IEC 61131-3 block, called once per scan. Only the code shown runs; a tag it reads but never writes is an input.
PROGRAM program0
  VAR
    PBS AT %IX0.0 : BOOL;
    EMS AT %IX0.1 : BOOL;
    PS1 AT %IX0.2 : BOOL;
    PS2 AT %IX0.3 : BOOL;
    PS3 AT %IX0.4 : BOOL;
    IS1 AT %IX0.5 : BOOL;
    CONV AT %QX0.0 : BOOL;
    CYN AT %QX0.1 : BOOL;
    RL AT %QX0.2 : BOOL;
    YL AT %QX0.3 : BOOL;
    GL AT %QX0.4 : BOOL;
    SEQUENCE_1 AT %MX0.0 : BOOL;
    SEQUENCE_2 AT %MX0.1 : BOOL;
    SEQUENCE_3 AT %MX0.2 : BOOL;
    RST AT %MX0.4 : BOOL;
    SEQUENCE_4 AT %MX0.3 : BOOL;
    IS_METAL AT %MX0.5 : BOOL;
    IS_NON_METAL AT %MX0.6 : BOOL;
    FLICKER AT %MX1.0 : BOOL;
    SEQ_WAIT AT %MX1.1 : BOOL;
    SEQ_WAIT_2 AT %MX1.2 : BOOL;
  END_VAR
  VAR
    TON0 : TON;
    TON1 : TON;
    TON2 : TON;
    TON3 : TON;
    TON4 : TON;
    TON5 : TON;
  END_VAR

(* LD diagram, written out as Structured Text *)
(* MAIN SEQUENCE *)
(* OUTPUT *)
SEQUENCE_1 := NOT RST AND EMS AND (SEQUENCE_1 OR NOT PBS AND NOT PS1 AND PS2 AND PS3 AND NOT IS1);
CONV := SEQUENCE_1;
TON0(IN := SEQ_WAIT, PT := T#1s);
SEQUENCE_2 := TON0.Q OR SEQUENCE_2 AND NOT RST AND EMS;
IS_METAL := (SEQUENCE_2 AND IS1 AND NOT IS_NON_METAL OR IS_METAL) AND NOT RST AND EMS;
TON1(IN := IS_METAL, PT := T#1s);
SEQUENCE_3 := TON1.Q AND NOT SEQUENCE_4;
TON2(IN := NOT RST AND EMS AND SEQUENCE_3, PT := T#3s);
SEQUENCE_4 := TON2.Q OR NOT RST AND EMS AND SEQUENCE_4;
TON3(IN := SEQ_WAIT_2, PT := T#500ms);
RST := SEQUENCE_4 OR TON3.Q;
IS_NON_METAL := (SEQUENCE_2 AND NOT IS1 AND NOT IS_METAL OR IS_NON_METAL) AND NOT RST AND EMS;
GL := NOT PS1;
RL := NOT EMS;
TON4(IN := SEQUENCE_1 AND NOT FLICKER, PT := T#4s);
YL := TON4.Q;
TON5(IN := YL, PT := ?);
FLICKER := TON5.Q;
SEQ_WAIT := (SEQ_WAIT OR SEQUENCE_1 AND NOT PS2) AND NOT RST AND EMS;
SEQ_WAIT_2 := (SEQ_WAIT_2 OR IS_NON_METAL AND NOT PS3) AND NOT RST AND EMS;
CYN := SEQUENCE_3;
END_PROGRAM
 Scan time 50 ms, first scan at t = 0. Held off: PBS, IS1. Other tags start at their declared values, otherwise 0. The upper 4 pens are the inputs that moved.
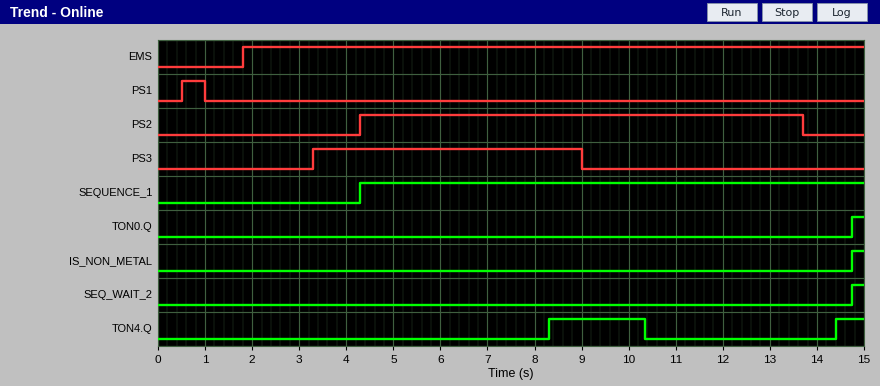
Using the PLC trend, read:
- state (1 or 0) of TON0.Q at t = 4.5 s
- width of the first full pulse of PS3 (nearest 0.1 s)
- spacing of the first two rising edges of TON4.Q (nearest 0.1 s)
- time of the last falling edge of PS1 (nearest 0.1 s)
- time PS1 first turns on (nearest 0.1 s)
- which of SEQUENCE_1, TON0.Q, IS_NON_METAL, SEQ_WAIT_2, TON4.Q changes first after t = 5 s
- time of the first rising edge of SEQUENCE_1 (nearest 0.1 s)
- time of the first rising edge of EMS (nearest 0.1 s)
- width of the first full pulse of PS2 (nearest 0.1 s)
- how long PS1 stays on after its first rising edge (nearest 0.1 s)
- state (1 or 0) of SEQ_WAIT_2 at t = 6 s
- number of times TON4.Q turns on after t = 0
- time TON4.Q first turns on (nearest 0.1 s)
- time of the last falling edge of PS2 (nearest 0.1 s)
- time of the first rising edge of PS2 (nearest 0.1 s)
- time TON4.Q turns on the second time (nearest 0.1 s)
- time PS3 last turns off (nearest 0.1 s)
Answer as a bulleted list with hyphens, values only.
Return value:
- 0
- 5.7 s
- 6.1 s
- 1.0 s
- 0.5 s
- TON4.Q
- 4.3 s
- 1.8 s
- 9.4 s
- 0.5 s
- 0
- 2
- 8.3 s
- 13.7 s
- 4.3 s
- 14.4 s
- 9.0 s
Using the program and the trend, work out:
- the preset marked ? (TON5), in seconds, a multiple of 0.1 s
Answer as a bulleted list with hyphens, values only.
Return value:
- 2.0 s
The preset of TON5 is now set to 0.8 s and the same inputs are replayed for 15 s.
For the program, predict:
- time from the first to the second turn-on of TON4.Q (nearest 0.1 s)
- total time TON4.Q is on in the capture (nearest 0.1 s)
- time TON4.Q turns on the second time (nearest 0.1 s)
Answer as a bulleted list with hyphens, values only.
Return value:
- 4.9 s
- 1.7 s
- 13.2 s
